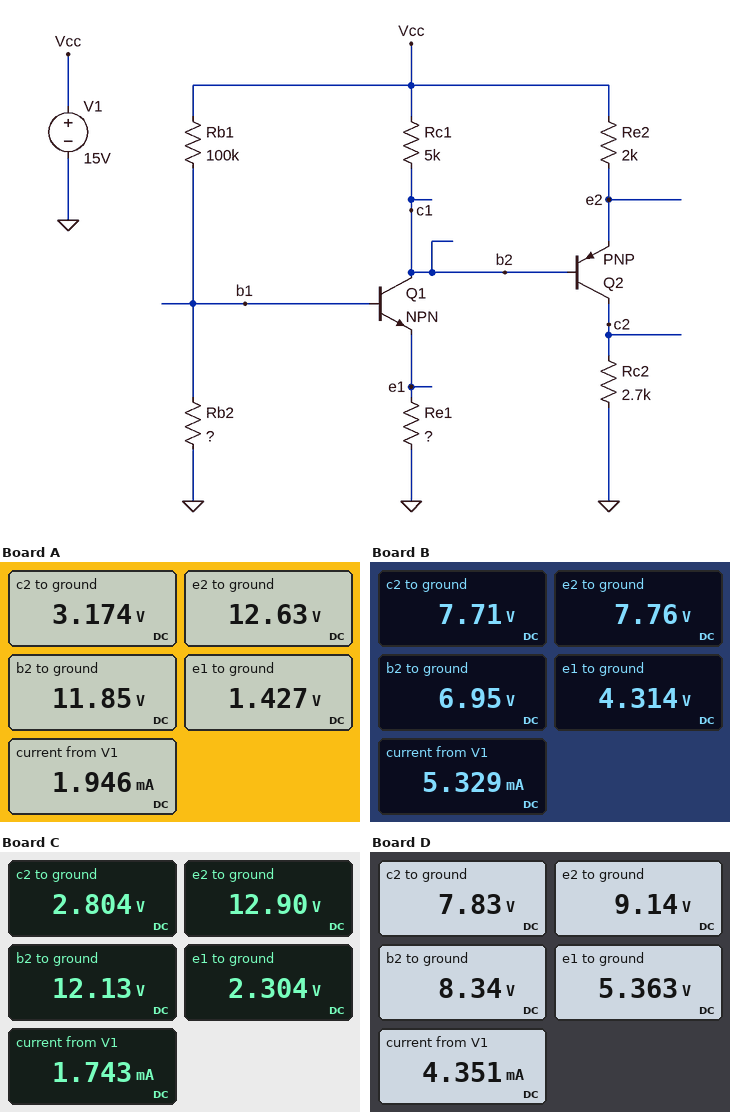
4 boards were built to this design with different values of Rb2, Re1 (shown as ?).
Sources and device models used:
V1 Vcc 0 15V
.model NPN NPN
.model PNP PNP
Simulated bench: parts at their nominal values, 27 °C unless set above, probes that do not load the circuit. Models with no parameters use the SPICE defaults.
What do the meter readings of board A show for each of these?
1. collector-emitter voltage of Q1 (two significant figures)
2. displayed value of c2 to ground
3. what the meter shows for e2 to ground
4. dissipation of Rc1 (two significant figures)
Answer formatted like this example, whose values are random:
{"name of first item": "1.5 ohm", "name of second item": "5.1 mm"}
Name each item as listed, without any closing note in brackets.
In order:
{"collector-emitter voltage of Q1": "10 V", "displayed value of c2 to ground": "3.174 V", "what the meter shows for e2 to ground": "12.63 V", "dissipation of Rc1": "2.0 mW"}
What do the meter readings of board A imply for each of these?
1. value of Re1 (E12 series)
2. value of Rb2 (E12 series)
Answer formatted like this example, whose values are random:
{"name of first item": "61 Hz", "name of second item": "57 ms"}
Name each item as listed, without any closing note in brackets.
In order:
{"value of Re1": "2.2 kΩ", "value of Rb2": "18 kΩ"}
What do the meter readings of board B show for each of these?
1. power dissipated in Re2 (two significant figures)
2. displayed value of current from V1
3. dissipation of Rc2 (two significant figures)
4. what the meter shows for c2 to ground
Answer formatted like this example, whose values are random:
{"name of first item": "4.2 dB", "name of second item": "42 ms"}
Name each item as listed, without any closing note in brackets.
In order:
{"power dissipated in Re2": "26 mW", "displayed value of current from V1": "5.329 mA", "dissipation of Rc2": "22 mW", "what the meter shows for c2 to ground": "7.71 V"}
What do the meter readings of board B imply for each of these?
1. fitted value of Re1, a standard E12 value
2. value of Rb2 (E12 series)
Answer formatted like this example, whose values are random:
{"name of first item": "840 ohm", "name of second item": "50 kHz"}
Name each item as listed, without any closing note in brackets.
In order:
{"fitted value of Re1, a standard E12 value": "1.8 kΩ", "value of Rb2": "68 kΩ"}
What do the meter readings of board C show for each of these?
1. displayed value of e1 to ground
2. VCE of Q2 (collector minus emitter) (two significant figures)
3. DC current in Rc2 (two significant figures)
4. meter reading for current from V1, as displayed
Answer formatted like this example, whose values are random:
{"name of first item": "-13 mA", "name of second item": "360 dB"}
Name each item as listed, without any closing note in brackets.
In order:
{"displayed value of e1 to ground": "2.304 V", "VCE of Q2 (collector minus emitter)": "-10 V", "DC current in Rc2": "1.0 mA", "meter reading for current from V1, as displayed": "1.743 mA"}
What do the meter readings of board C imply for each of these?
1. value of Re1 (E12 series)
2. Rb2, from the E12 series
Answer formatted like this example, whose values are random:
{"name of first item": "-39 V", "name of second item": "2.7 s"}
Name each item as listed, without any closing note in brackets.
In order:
{"value of Re1": "3.9 kΩ", "Rb2, from the E12 series": "27 kΩ"}
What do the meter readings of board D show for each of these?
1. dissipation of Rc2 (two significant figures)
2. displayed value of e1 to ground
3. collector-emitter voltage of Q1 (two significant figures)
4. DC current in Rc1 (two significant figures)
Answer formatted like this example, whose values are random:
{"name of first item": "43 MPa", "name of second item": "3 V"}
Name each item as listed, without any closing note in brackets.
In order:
{"dissipation of Rc2": "23 mW", "displayed value of e1 to ground": "5.363 V", "collector-emitter voltage of Q1": "3.0 V", "DC current in Rc1": "1.3 mA"}
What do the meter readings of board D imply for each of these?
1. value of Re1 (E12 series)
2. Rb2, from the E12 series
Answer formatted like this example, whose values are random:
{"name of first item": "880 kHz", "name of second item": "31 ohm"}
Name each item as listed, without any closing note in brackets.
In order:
{"value of Re1": "3.9 kΩ", "Rb2, from the E12 series": "82 kΩ"}
